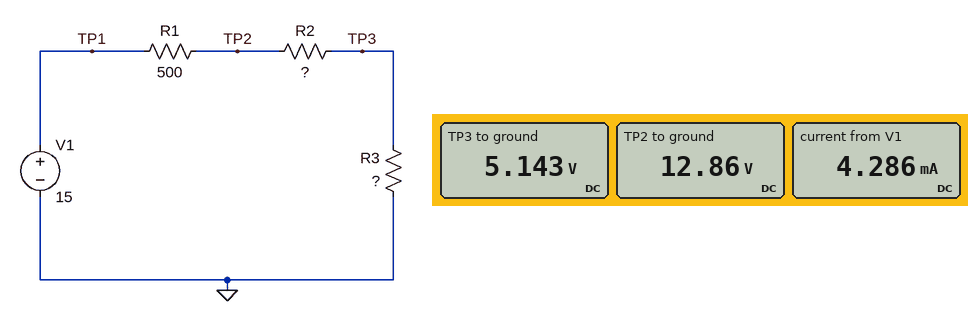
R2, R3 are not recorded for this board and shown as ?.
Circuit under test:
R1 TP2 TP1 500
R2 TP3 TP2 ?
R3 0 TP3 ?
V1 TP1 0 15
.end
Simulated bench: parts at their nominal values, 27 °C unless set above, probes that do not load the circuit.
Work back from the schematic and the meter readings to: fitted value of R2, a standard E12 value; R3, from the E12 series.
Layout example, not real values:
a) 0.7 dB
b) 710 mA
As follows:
a) 1.8 kΩ
b) 1.2 kΩ
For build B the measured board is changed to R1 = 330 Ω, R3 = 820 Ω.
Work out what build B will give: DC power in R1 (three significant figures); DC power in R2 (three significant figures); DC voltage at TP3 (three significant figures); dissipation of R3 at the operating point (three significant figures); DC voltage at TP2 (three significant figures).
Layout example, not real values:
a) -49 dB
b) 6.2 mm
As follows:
a) 8.53 mW
b) 46.5 mW
c) 4.17 V
d) 21.2 mW
e) 13.3 V
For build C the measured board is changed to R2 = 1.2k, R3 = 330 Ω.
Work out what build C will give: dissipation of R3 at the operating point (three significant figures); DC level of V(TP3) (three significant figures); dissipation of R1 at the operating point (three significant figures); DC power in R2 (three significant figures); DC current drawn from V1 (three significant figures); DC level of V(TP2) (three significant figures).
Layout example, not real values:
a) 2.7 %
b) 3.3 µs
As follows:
a) 18.0 mW
b) 2.44 V
c) 27.3 mW
d) 65.5 mW
e) 7.39 mA
f) 11.3 V
